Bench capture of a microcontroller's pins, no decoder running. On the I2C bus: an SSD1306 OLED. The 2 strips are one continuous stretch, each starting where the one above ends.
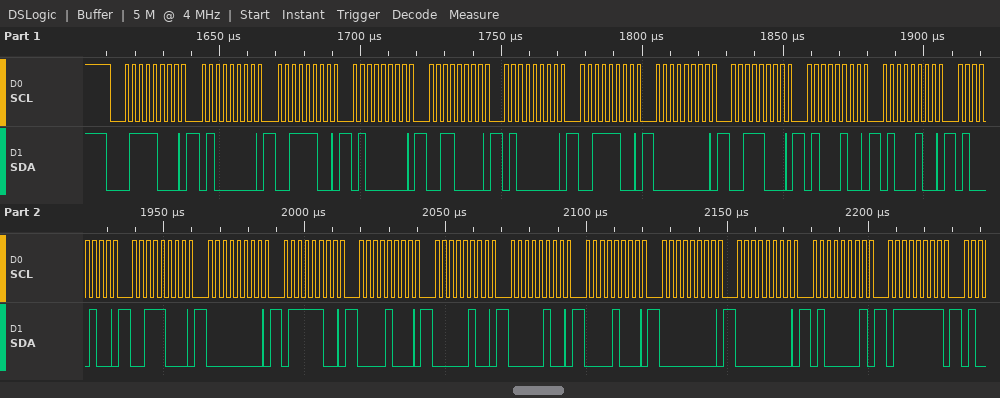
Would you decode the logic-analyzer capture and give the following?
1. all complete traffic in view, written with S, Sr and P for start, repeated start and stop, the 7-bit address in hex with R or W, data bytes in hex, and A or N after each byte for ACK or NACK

S 3CW A 40 A 3C A 40 A 30 A 40 A 3C A 00 A 38 A 44 A 44 A 44 A 38 A 00 A 7C A 08 A 04 A 04 A 08 A 00 A 00 A 41 A 7F A
